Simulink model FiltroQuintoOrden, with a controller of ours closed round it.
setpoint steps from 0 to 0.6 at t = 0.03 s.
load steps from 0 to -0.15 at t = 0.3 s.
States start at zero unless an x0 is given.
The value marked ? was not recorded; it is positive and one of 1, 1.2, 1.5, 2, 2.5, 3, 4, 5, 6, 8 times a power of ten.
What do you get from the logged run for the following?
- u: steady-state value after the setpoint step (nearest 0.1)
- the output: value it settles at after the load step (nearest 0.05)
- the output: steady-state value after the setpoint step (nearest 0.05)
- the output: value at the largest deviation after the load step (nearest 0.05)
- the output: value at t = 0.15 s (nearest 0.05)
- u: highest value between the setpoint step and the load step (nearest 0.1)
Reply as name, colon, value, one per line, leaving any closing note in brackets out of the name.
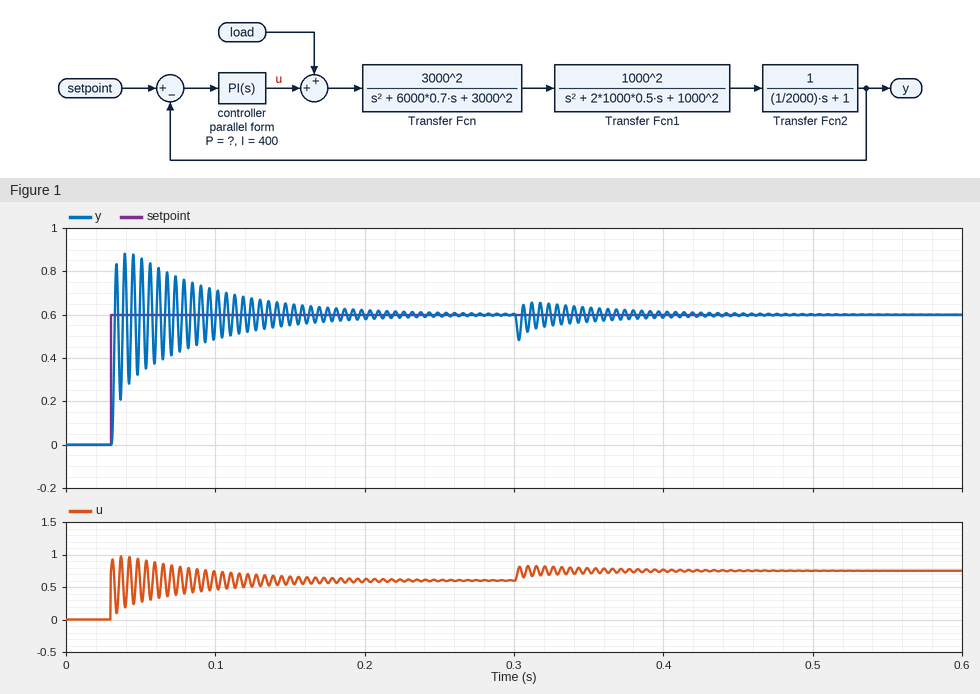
u: steady-state value after the setpoint step: 0.6
the output: value it settles at after the load step: 0.60
the output: steady-state value after the setpoint step: 0.60
the output: value at the largest deviation after the load step: 0.50
the output: value at t = 0.15 s: 0.55
u: highest value between the setpoint step and the load step: 1.0
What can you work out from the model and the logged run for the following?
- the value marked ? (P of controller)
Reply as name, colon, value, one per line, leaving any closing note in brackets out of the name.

the value marked ?: 1.2
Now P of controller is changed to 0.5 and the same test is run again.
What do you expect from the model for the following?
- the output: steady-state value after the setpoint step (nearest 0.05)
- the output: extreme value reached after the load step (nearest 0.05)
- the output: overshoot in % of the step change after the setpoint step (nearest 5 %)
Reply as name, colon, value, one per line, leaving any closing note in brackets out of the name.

the output: steady-state value after the setpoint step: 0.60
the output: extreme value reached after the load step: 0.45
the output: overshoot in % of the step change after the setpoint step: 20 %
